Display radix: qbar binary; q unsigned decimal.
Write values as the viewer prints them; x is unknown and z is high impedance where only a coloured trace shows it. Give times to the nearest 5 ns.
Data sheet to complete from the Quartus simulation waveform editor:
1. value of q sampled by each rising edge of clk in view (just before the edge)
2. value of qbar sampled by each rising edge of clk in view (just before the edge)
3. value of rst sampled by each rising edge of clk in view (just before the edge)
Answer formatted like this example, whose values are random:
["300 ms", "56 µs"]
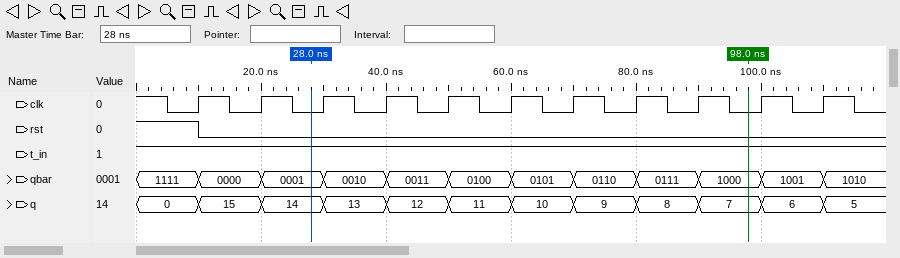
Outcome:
["0, 15, 14, 13, 12, 11, 10, 9, 8, 7, 6", "1111, 0000, 0001, 0010, 0011, 0100, 0101, 0110, 0111, 1000, 1001", "1 0 0 0 0 0 0 0 0 0 0"]
